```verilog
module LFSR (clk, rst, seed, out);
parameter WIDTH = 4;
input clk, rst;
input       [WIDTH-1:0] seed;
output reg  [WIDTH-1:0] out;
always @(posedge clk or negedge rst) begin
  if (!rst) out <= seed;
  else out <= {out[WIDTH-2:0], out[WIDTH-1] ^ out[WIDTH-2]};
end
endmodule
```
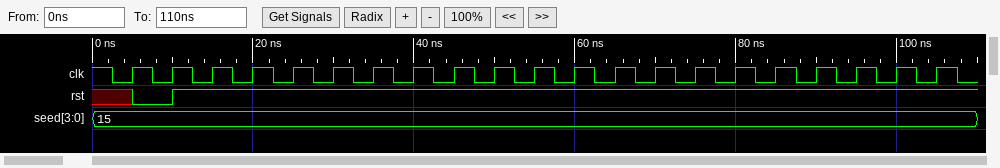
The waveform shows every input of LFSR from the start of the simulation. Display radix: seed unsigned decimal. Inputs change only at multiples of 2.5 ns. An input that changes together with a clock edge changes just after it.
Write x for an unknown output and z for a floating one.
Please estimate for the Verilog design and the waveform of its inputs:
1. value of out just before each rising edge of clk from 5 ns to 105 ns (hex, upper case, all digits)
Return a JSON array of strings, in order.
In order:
["x, F, F, E, C, 8, 1, 2, 4, 9, 3, 6, D, A, 5, B, 7, F, E, C, 8"]
